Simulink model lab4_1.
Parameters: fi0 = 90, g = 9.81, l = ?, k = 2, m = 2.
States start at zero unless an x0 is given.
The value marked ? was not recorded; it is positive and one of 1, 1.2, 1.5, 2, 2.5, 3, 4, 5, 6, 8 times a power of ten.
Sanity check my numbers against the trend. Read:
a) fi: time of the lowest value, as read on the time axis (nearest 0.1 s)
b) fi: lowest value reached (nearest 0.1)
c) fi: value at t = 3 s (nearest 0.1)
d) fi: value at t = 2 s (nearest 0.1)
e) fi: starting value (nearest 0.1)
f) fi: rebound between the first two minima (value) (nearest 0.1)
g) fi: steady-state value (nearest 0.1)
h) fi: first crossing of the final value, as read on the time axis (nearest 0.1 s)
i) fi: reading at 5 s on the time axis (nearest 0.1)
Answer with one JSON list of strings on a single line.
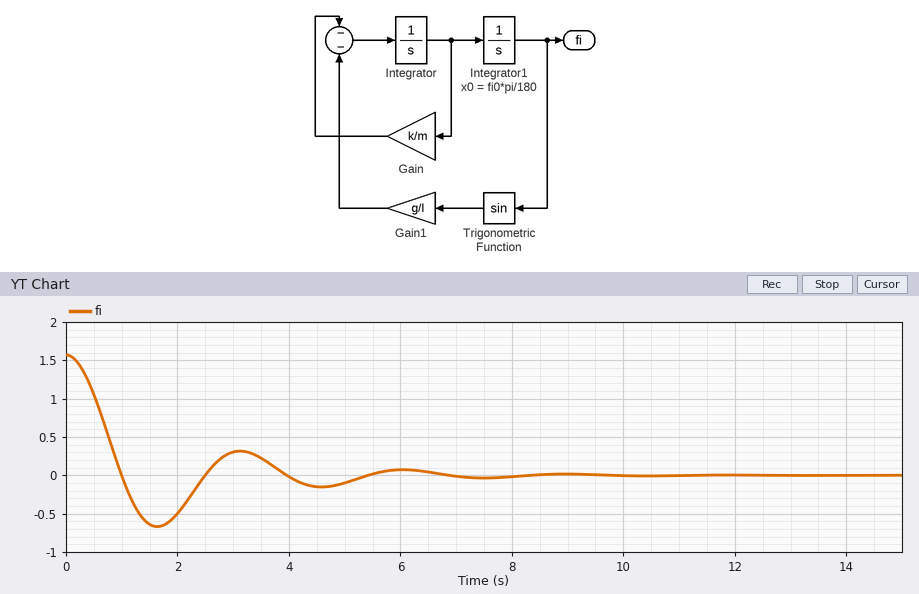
["1.6 s", "-0.7", "0.3", "-0.5", "1.6", "0.3", "0.0", "1.0 s", "-0.1"]
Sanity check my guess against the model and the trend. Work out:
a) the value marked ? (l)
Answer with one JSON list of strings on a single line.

["2"]
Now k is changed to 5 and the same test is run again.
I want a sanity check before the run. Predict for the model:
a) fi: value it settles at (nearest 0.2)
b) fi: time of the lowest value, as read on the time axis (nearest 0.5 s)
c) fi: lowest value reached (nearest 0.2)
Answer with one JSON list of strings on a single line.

["0.0", "2.0 s", "-0.2"]
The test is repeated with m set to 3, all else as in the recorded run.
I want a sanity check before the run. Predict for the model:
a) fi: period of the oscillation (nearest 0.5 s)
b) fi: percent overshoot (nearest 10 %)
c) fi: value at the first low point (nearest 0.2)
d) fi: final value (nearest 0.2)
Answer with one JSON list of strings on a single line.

["3.0 s", "60 %", "-0.8", "0.0"]
